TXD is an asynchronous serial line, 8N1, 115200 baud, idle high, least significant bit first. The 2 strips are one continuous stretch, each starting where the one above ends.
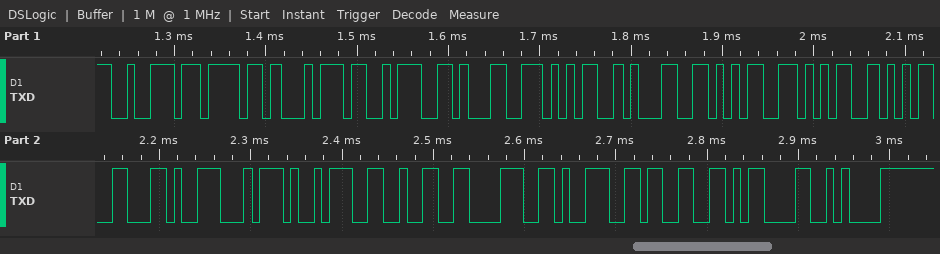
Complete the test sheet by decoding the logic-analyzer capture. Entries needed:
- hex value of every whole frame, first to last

0x72 0x6F 0x74 0x3A 0x31 0x35 0x31 0x35 0x35 0x35 0x2C 0x74 0x3A 0x32 0x38 0x39 0x33 0x0D 0x0A
